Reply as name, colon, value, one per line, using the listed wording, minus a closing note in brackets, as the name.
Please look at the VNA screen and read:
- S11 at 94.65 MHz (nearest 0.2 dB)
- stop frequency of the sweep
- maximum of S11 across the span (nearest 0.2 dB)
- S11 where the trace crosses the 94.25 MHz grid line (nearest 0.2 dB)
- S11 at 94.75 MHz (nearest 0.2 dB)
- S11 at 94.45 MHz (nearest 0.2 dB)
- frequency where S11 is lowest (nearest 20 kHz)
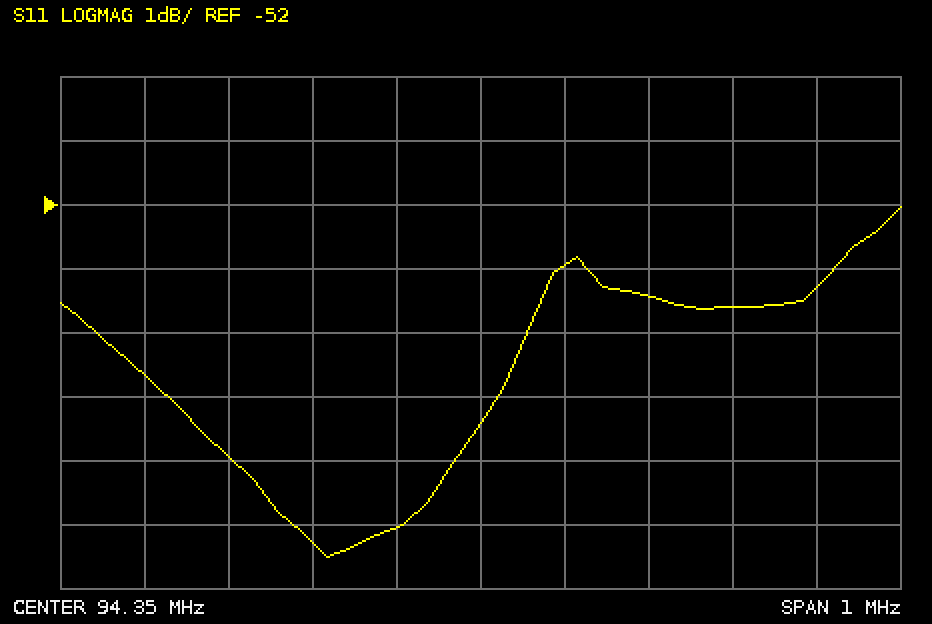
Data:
S11 at 94.65 MHz: -53.6 dB
stop frequency of the sweep: 94.85 MHz
maximum of S11 across the span: -52.0 dB
S11 where the trace crosses the 94.25 MHz grid line: -57.0 dB
S11 at 94.75 MHz: -53.2 dB
S11 at 94.45 MHz: -53.0 dB
frequency where S11 is lowest: 94.16 MHz
